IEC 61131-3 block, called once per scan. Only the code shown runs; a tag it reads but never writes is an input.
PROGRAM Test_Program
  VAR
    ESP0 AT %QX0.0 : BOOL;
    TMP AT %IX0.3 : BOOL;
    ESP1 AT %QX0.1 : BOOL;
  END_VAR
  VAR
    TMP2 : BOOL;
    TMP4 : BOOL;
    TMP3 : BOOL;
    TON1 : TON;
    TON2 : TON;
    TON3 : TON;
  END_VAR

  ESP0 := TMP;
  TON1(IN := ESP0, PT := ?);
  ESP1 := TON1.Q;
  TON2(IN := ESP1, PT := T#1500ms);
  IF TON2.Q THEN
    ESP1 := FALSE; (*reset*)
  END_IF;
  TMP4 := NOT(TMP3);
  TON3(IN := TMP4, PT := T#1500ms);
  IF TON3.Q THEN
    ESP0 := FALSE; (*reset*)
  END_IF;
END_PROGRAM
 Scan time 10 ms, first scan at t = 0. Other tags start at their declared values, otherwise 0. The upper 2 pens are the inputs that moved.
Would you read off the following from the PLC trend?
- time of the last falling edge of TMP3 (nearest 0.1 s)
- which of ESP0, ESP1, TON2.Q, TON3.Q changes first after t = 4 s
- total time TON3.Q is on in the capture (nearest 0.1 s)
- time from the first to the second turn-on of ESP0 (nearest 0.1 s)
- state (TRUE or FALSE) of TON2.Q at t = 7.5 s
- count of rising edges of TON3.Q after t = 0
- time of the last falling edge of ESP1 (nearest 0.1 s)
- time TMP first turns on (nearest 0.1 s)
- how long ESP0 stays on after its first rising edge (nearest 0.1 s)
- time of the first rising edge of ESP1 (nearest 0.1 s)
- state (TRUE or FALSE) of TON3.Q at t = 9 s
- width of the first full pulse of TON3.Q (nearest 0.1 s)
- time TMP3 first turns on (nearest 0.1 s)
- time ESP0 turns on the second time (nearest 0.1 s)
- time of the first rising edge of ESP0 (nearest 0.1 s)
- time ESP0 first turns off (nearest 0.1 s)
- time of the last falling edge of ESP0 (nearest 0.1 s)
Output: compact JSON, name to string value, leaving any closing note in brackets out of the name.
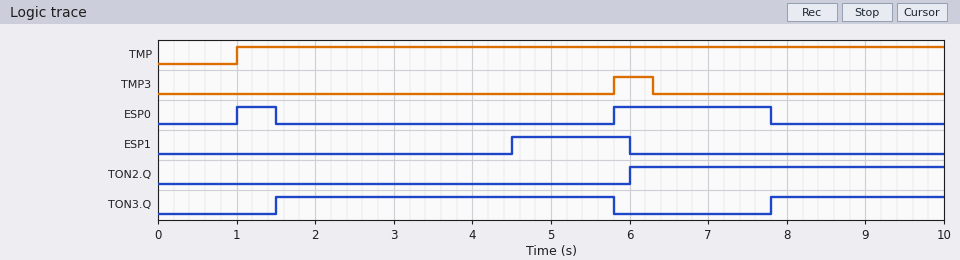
{"time of the last falling edge of TMP3": "6.3 s", "which of ESP0, ESP1, TON2.Q, TON3.Q changes first after t = 4 s": "ESP1", "total time TON3.Q is on in the capture": "6.5 s", "time from the first to the second turn-on of ESP0": "4.8 s", "state (TRUE or FALSE) of TON2.Q at t = 7.5 s": "TRUE", "count of rising edges of TON3.Q after t = 0": "2", "time of the last falling edge of ESP1": "6.0 s", "time TMP first turns on": "1.0 s", "how long ESP0 stays on after its first rising edge": "0.5 s", "time of the first rising edge of ESP1": "4.5 s", "state (TRUE or FALSE) of TON3.Q at t = 9 s": "TRUE", "width of the first full pulse of TON3.Q": "4.3 s", "time TMP3 first turns on": "5.8 s", "time ESP0 turns on the second time": "5.8 s", "time of the first rising edge of ESP0": "1.0 s", "time ESP0 first turns off": "1.5 s", "time of the last falling edge of ESP0": "7.8 s"}
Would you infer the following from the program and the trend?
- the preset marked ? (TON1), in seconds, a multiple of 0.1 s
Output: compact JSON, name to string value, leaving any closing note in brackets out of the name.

{"the preset marked ? (TON1), in seconds, a multiple of 0.1 s": "3.5 s"}
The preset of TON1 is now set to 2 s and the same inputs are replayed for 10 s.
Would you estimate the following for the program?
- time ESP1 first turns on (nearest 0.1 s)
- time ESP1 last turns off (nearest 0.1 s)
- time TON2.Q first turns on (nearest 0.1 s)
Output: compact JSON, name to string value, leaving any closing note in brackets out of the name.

{"time ESP1 first turns on": "3.0 s", "time ESP1 last turns off": "4.5 s", "time TON2.Q first turns on": "4.5 s"}
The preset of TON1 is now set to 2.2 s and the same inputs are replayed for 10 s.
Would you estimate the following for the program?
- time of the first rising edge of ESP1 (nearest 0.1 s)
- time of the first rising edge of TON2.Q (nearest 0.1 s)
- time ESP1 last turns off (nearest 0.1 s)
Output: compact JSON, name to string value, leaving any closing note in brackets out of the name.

{"time of the first rising edge of ESP1": "3.2 s", "time of the first rising edge of TON2.Q": "4.7 s", "time ESP1 last turns off": "4.7 s"}
